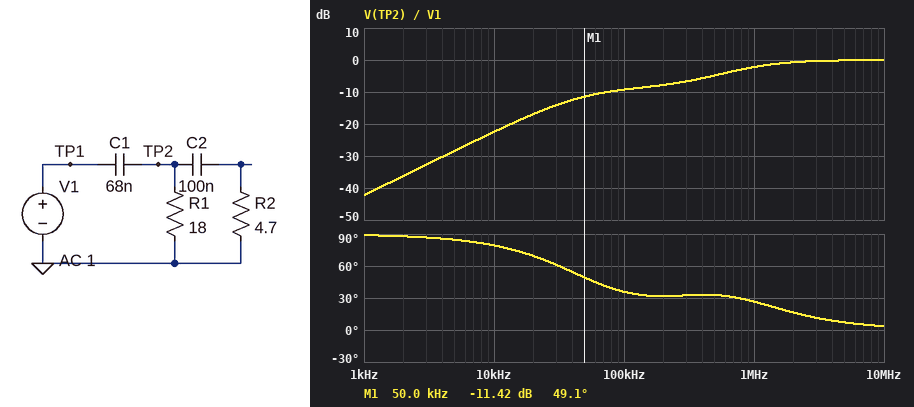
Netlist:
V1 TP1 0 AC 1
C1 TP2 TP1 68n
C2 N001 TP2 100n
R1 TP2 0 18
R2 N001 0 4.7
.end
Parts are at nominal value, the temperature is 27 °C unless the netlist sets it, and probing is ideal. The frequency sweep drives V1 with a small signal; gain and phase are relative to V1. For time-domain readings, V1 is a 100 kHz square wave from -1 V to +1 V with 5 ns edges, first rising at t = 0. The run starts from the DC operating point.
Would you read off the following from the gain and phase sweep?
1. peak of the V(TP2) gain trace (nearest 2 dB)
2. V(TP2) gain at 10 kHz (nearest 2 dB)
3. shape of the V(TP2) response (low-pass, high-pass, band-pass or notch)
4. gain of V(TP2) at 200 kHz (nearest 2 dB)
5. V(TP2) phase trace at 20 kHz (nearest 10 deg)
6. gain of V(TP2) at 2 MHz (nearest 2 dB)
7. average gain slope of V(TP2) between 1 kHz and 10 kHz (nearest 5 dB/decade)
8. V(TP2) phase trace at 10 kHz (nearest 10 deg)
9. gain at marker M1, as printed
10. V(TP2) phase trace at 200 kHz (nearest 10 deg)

0 dB
-22 dB
high-pass
-8 dB
70 deg
0 dB
20 dB/decade
80 deg
-11.42 dB
30 deg
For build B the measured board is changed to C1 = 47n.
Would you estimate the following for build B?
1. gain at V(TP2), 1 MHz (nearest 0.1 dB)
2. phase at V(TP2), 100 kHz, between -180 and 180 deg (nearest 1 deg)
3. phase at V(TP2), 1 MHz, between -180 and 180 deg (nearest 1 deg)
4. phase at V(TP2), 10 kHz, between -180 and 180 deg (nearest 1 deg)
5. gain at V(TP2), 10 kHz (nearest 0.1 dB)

-3.4 dB
40 deg
34 deg
81 deg
-25.6 dB
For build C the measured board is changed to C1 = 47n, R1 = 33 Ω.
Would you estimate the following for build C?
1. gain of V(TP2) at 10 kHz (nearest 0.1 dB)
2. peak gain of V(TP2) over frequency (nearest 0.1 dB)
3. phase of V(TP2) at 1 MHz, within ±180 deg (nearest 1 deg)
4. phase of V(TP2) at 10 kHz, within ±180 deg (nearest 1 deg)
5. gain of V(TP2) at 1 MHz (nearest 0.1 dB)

-20.7 dB
0 dB
32 deg
73 deg
-3.1 dB
